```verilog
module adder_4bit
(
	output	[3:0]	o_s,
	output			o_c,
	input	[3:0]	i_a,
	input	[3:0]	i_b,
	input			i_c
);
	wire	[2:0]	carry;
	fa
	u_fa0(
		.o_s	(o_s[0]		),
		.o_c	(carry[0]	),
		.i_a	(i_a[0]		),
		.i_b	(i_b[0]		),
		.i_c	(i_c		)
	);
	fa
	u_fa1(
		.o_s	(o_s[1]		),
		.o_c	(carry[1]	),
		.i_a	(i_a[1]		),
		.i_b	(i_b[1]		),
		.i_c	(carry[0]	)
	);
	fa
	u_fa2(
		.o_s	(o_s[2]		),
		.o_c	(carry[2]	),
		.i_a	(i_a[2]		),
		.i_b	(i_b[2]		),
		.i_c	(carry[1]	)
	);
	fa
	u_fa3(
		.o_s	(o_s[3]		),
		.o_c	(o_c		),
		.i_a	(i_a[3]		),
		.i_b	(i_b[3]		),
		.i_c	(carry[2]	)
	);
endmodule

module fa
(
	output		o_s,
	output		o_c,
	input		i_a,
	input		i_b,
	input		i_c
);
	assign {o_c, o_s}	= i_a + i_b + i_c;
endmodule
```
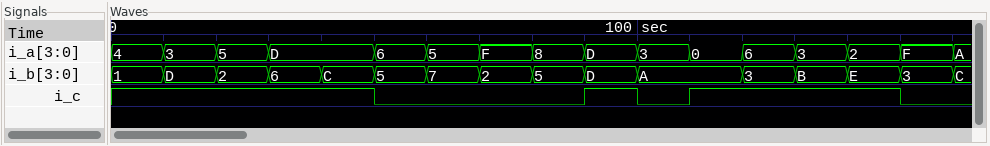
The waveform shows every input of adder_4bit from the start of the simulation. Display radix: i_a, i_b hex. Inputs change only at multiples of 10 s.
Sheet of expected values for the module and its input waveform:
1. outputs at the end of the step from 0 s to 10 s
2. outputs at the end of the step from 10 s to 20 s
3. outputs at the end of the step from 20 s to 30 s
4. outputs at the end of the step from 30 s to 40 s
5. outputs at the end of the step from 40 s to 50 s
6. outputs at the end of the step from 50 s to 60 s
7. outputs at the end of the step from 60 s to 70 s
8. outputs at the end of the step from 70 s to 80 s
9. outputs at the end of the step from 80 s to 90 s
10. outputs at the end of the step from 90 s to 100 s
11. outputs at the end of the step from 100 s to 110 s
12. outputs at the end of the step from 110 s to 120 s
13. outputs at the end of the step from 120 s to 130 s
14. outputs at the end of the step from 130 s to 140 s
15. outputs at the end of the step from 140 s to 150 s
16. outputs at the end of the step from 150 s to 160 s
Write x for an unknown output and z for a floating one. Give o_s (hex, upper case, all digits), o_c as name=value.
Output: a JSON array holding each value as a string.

["o_s=6, o_c=0", "o_s=1, o_c=1", "o_s=8, o_c=0", "o_s=4, o_c=1", "o_s=A, o_c=1", "o_s=B, o_c=0", "o_s=C, o_c=0", "o_s=1, o_c=1", "o_s=D, o_c=0", "o_s=B, o_c=1", "o_s=D, o_c=0", "o_s=B, o_c=0", "o_s=A, o_c=0", "o_s=F, o_c=0", "o_s=1, o_c=1", "o_s=2, o_c=1"]
